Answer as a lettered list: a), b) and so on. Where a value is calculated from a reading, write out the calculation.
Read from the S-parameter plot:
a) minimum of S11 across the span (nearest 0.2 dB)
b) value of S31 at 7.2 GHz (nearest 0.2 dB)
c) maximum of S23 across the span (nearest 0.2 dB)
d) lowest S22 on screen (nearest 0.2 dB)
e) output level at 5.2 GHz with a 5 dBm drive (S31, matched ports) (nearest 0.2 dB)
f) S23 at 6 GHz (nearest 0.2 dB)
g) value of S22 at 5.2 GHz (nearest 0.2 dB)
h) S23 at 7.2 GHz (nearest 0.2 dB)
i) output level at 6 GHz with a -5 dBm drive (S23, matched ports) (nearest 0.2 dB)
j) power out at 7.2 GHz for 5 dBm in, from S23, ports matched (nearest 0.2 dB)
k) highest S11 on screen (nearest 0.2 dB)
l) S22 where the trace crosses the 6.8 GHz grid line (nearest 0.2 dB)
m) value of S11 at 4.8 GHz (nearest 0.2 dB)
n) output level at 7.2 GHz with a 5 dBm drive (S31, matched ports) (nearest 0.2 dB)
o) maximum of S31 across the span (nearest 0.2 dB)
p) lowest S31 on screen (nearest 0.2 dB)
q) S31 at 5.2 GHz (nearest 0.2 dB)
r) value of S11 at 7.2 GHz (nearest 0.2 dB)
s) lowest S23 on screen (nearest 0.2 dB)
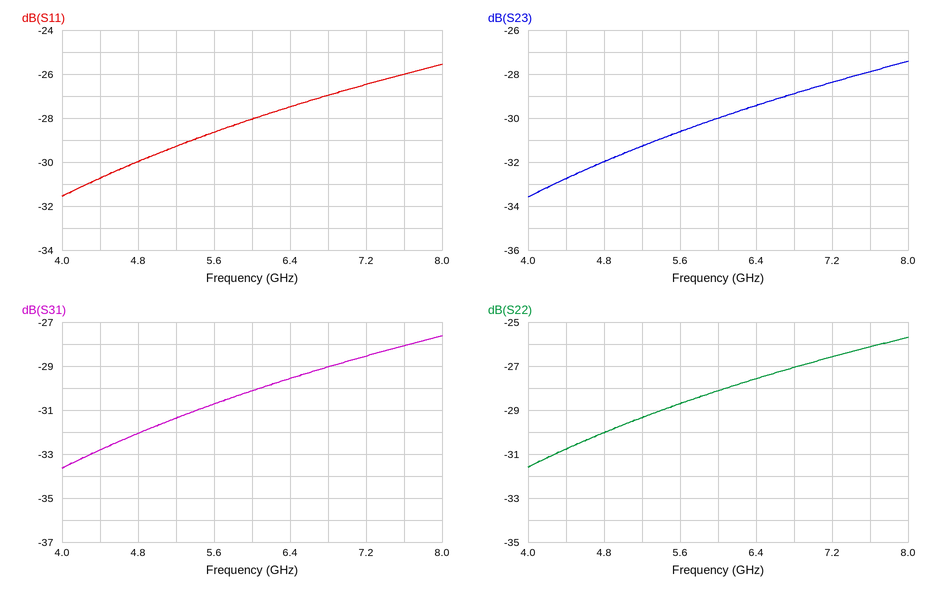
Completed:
a) -31.6 dB
b) -28.6 dB
c) -27.4 dB
d) -31.6 dB
e) 5 dBm + (-31.4 dB) = -26.4 dBm
f) -30.0 dB
g) -29.4 dB
h) -28.4 dB
i) -5 dBm + (-30.0 dB) = -35.0 dBm
j) 5 dBm + (-28.4 dB) = -23.4 dBm
k) -25.6 dB
l) -27.0 dB
m) -30.0 dB
n) 5 dBm + (-28.6 dB) = -23.6 dBm
o) -27.6 dB
p) -33.6 dB
q) -31.4 dB
r) -26.4 dB
s) -33.6 dB
